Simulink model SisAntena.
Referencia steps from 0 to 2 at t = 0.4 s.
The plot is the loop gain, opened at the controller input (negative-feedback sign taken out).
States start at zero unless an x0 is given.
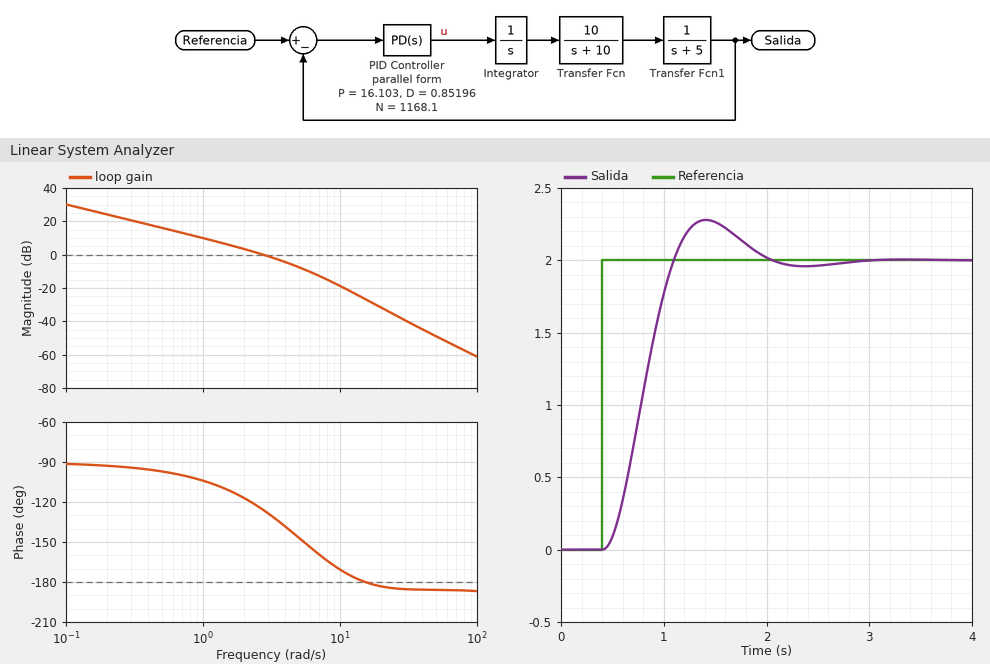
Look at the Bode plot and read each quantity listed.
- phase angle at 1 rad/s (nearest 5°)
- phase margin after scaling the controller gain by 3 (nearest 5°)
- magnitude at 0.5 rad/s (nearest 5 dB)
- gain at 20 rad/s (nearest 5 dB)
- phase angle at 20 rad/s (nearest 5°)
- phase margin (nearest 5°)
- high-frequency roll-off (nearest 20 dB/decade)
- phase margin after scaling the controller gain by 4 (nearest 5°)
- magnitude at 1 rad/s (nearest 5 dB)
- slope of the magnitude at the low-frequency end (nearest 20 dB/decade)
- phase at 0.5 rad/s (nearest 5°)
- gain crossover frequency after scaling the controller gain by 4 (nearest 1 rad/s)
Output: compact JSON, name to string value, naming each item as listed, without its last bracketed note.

{"phase angle at 1 rad/s": "-105°", "phase margin after scaling the controller gain by 3": "30°", "magnitude at 0.5 rad/s": "15 dB", "gain at 20 rad/s": "-30 dB", "phase angle at 20 rad/s": "-185°", "phase margin": "55°", "high-frequency roll-off": "-40 dB/decade", "phase margin after scaling the controller gain by 4": "20°", "magnitude at 1 rad/s": "10 dB", "slope of the magnitude at the low-frequency end": "-20 dB/decade", "phase at 0.5 rad/s": "-95°", "gain crossover frequency after scaling the controller gain by 4": "7 rad/s"}
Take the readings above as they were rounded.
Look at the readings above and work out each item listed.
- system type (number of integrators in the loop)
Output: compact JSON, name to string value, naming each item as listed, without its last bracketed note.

{"system type": "1"}
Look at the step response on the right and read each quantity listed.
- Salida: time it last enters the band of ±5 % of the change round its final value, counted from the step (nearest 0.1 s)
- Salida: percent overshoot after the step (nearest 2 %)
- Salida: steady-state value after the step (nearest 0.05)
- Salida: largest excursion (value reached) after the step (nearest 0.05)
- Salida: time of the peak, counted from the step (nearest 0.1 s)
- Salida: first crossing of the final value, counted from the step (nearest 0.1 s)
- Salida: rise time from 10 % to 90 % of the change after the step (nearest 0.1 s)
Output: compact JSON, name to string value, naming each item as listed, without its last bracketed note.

{"Salida: time it last enters the band of ±5 % of the change round its final value, counted from the step": "1.4 s", "Salida: percent overshoot after the step": "14 %", "Salida: steady-state value after the step": "2.00", "Salida: largest excursion (value reached) after the step": "2.30", "Salida: time of the peak, counted from the step": "1.0 s", "Salida: first crossing of the final value, counted from the step": "0.7 s", "Salida: rise time from 10 % to 90 % of the change after the step": "0.5 s"}
